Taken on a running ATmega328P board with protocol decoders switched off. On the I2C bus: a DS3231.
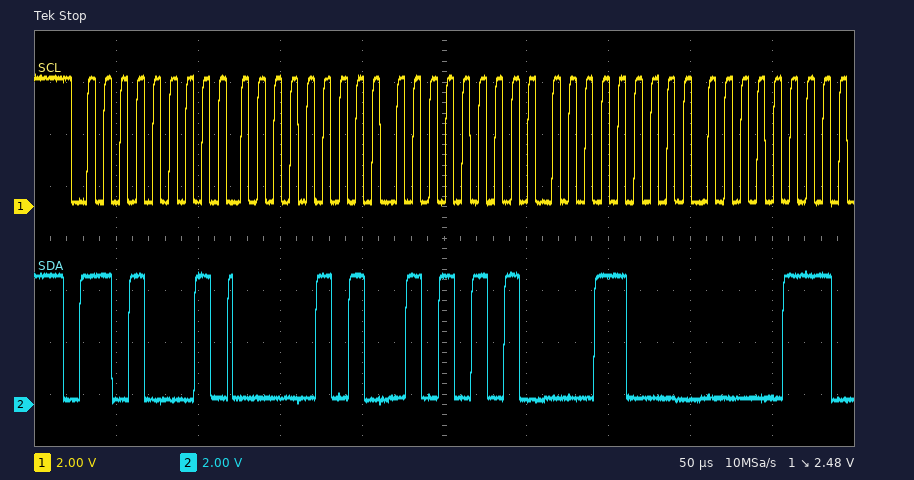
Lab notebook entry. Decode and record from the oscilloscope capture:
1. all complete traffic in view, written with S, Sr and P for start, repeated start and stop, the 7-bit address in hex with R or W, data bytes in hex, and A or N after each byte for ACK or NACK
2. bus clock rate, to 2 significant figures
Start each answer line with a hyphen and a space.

- S 68R A 05 A 55 A 18 A 07 A
- 100 kHz
